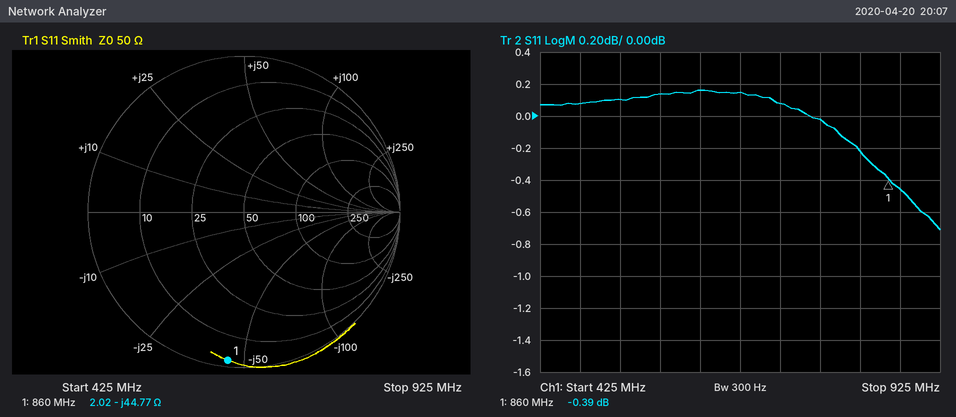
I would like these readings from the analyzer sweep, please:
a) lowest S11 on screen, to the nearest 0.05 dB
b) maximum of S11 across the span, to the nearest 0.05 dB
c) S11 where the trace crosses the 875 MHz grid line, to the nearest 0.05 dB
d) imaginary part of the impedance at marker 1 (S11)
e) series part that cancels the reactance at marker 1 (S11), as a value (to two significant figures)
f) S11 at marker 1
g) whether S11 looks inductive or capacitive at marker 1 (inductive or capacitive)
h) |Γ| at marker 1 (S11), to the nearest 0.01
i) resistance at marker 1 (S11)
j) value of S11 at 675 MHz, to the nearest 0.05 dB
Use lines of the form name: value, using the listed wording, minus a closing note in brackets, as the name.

lowest S11 on screen, to the nearest 0.05 dB: -0.70 dB
maximum of S11 across the span, to the nearest 0.05 dB: 0.15 dB
S11 where the trace crosses the 875 MHz grid line, to the nearest 0.05 dB: -0.45 dB
imaginary part of the impedance at marker 1: -44.77 Ω
series part that cancels the reactance at marker 1 (S11), as a value: 8.3 nH
S11 at marker 1: -0.39 dB
whether S11 looks inductive or capacitive at marker 1: capacitive
|Γ| at marker 1 (S11), to the nearest 0.01: 0.96
resistance at marker 1: 2.02 Ω
value of S11 at 675 MHz, to the nearest 0.05 dB: 0.15 dB
